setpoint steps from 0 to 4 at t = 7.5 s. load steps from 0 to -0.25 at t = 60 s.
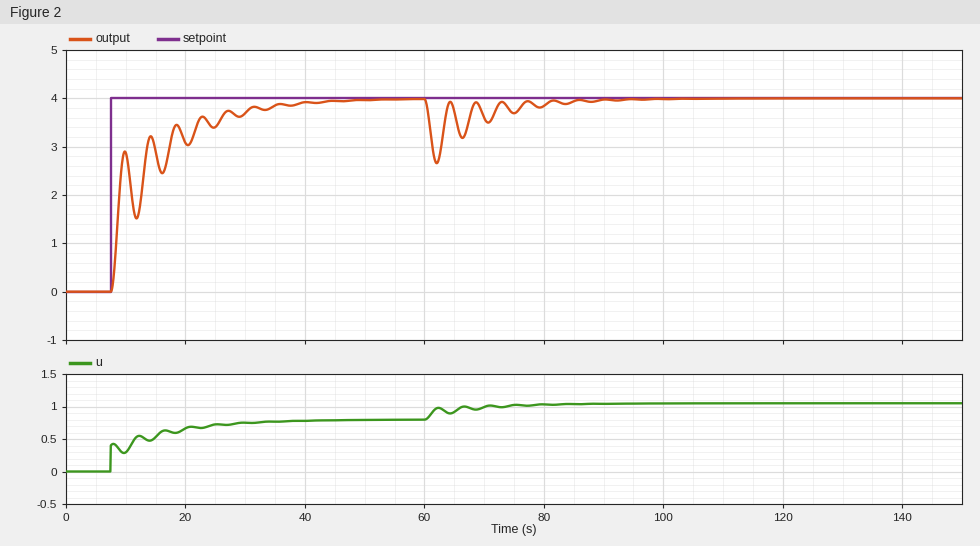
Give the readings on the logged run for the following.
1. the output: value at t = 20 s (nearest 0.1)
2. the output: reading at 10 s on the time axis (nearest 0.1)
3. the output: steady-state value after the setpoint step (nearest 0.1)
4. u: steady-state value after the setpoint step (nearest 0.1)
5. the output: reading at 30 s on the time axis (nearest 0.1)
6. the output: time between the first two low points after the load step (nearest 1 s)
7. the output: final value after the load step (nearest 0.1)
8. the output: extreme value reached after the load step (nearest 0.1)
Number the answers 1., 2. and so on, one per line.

1. 3.1
2. 2.9
3. 4.0
4. 0.8
5. 3.7
6. 4 s
7. 4.0
8. 2.7
